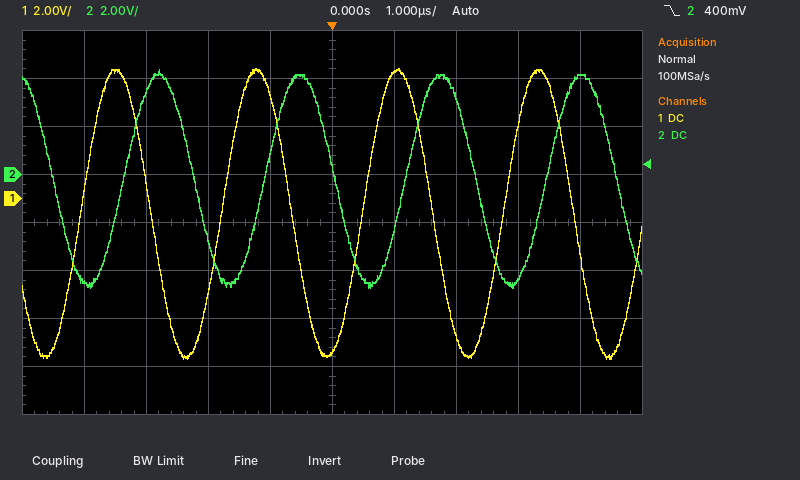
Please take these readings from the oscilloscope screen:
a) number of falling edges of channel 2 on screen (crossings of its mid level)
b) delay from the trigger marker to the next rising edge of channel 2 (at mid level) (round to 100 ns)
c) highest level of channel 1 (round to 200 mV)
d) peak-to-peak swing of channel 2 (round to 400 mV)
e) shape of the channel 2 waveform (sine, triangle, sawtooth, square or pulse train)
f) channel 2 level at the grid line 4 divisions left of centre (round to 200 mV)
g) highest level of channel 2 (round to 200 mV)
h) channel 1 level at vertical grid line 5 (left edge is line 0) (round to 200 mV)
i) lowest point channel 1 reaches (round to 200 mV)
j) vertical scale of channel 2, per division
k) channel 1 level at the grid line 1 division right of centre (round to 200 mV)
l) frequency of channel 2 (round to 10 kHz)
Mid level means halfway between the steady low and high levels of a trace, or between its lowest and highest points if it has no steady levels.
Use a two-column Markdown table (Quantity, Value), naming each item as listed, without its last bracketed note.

| Quantity | Value |
|---|---|
| number of falling edges of channel 2 on screen | 5 |
| delay from the trigger marker to the next rising edge of channel 2 (at mid level) | 1.2 µs |
| highest level of channel 1 | 5.4 V |
| peak-to-peak swing of channel 2 | 9.2 V |
| shape of the channel 2 waveform | sine |
| channel 2 level at the grid line 4 divisions left of centre | -4.4 V |
| highest level of channel 2 | 4.4 V |
| channel 1 level at vertical grid line 5 (left edge is line 0) | -6.4 V |
| lowest point channel 1 reaches | -6.6 V |
| vertical scale of channel 2, per division | 2 V |
| channel 1 level at the grid line 1 division right of centre | 5.2 V |
| frequency of channel 2 | 440 kHz |
